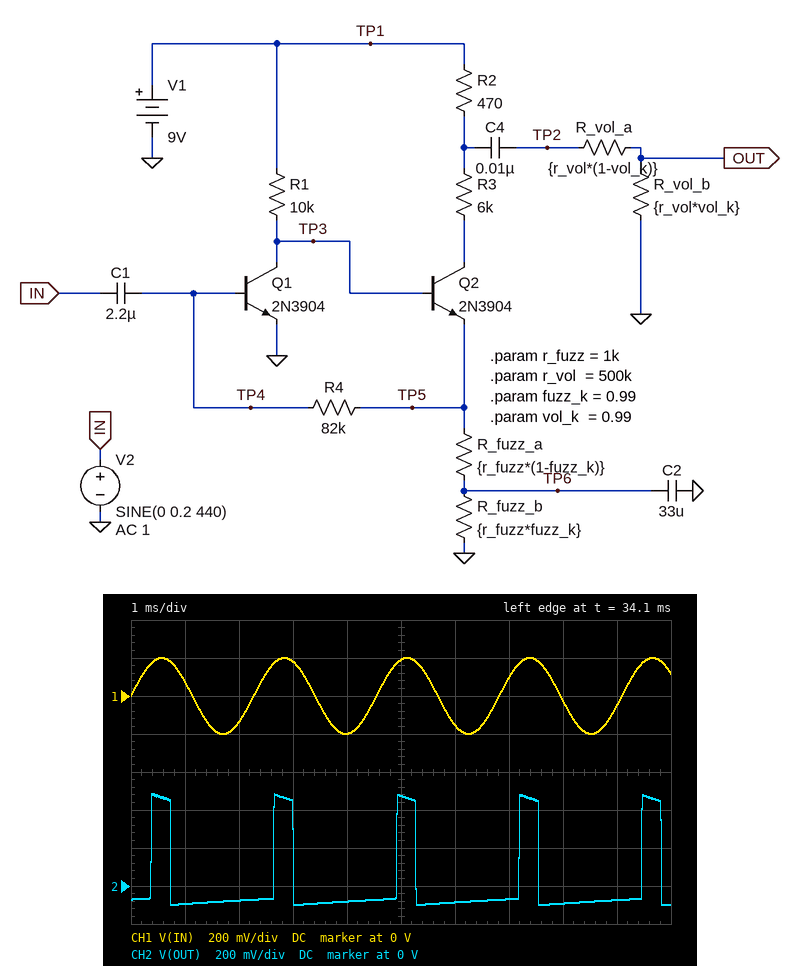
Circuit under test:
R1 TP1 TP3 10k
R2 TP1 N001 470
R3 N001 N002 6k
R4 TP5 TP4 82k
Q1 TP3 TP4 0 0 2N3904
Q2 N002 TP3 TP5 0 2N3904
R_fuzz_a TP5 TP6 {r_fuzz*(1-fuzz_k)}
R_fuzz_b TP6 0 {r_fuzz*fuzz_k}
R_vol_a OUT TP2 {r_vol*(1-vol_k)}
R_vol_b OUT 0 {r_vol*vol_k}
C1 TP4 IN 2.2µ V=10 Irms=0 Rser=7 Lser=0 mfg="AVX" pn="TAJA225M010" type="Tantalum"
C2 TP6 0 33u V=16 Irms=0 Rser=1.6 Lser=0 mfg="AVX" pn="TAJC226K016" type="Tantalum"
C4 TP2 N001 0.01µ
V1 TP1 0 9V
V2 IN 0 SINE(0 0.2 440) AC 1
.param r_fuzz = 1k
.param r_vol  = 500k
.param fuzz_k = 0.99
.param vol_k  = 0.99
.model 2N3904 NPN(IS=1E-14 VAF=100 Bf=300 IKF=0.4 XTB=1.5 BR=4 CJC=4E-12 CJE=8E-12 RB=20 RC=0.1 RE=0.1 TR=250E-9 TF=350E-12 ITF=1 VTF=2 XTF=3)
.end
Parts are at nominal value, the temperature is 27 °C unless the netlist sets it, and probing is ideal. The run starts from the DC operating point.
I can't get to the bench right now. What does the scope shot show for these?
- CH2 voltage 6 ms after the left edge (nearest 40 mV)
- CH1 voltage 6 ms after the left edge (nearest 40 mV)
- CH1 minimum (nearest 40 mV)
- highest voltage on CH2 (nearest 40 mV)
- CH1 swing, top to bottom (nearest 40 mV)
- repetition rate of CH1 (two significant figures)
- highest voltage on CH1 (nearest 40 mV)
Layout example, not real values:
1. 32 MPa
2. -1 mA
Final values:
1. -80 mV
2. -160 mV
3. -200 mV
4. 480 mV
5. 400 mV
6. 440 Hz
7. 200 mV
